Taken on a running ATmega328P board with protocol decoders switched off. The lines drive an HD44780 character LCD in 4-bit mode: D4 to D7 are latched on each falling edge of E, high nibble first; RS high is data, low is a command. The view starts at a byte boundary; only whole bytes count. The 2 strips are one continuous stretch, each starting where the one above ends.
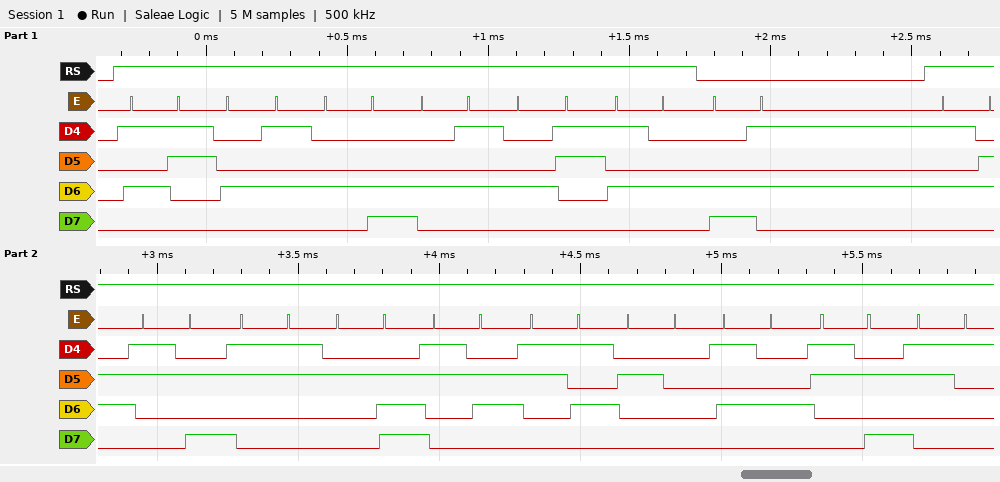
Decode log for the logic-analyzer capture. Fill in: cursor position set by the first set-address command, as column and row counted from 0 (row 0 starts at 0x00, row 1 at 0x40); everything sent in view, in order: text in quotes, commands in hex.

column 5, row 1
"SELECT" 0xC5 "V:3.65 T:1"
